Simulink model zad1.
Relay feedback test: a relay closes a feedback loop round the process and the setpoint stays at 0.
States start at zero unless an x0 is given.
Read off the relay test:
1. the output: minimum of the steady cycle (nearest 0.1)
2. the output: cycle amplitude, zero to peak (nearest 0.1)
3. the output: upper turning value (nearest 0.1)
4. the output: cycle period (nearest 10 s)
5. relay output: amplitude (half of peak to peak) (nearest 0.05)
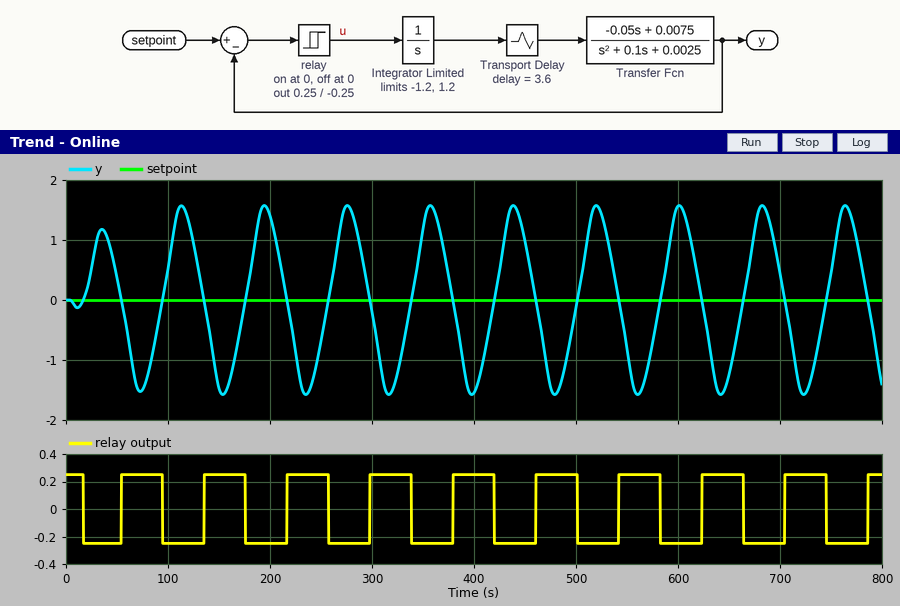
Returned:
-1.6
1.6
1.6
80 s
0.25
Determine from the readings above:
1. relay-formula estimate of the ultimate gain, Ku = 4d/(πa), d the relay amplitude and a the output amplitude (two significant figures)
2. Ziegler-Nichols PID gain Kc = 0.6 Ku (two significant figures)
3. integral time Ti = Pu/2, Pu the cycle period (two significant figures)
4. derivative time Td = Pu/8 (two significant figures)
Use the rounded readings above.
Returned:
0.20
0.12
40 s
10 s
